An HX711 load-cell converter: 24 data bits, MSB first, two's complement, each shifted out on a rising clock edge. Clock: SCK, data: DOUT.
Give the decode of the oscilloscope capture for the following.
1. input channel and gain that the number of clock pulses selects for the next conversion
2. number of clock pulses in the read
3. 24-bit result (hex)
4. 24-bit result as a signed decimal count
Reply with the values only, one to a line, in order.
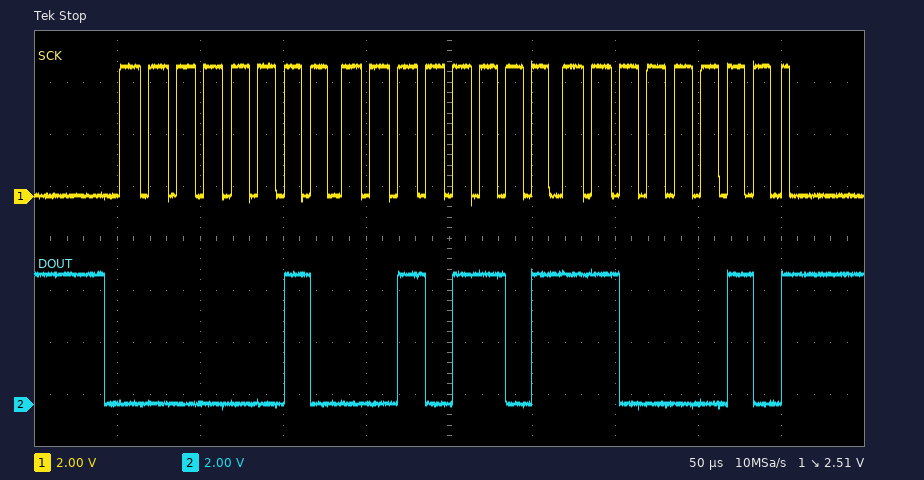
channel A, gain 128
25
0x022DC2
142786
